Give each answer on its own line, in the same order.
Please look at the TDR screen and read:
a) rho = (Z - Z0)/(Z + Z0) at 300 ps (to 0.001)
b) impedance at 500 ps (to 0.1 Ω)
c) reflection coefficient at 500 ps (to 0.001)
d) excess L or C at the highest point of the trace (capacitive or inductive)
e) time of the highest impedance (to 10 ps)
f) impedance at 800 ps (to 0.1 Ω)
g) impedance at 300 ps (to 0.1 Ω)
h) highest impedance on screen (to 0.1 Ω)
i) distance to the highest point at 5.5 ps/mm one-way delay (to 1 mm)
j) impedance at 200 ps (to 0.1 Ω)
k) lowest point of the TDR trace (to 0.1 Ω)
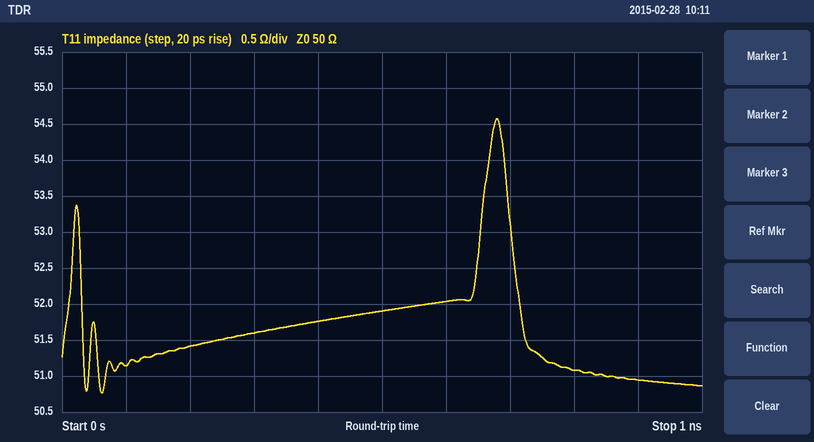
+0.016
51.9 Ω
+0.019
inductive
680 ps
51.1 Ω
51.6 Ω
54.6 Ω
62 mm
51.4 Ω
50.8 Ω
